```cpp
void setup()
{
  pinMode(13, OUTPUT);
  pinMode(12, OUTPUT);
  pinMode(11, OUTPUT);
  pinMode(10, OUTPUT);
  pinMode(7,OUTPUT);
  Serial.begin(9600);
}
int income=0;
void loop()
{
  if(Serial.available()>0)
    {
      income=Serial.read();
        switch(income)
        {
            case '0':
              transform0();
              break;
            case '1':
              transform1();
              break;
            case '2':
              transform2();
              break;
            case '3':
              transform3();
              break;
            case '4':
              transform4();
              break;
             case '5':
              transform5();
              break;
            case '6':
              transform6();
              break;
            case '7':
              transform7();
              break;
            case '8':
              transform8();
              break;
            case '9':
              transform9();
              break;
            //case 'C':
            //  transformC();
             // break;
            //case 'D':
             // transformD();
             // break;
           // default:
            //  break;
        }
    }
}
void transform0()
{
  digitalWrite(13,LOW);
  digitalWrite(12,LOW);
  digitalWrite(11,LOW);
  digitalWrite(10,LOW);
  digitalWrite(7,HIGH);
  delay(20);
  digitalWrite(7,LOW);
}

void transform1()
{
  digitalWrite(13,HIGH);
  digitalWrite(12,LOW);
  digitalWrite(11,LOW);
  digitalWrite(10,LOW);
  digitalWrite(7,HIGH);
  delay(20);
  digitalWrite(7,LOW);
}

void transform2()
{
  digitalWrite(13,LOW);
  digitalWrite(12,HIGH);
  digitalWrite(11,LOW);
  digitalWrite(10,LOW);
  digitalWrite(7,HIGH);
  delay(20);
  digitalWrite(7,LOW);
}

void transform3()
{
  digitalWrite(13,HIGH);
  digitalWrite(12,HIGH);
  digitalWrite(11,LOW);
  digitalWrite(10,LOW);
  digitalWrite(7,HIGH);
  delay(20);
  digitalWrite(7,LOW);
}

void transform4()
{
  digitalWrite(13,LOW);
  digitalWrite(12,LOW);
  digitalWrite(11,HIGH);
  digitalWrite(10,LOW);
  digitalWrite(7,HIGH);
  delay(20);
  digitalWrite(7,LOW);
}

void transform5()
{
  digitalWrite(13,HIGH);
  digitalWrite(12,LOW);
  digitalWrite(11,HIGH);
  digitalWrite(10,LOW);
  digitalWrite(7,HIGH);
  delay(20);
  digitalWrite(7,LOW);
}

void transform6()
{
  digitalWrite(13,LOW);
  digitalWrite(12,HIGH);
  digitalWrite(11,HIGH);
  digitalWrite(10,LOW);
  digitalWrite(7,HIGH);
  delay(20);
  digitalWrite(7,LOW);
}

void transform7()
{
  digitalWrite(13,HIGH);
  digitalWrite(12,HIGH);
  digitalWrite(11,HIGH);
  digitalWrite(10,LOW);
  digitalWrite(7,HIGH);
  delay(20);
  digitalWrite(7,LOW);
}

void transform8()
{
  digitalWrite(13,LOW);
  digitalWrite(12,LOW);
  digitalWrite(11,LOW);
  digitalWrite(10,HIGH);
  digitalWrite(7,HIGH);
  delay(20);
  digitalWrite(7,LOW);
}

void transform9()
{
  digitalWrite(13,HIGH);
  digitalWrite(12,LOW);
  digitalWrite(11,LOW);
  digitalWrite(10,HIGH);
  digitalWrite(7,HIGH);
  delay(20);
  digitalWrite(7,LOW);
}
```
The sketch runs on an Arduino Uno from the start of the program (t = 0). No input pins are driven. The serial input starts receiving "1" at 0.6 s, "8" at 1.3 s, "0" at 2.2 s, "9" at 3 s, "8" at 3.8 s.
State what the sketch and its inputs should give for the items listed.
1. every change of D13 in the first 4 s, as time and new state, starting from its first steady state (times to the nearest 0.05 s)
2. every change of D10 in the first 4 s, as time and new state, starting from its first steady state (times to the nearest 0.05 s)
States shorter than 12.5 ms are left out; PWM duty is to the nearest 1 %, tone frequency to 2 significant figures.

0 s low; 0.6 s high; 1.3 s low; 3 s high; 3.8 s low
0 s low; 1.3 s high; 2.2 s low; 3 s high
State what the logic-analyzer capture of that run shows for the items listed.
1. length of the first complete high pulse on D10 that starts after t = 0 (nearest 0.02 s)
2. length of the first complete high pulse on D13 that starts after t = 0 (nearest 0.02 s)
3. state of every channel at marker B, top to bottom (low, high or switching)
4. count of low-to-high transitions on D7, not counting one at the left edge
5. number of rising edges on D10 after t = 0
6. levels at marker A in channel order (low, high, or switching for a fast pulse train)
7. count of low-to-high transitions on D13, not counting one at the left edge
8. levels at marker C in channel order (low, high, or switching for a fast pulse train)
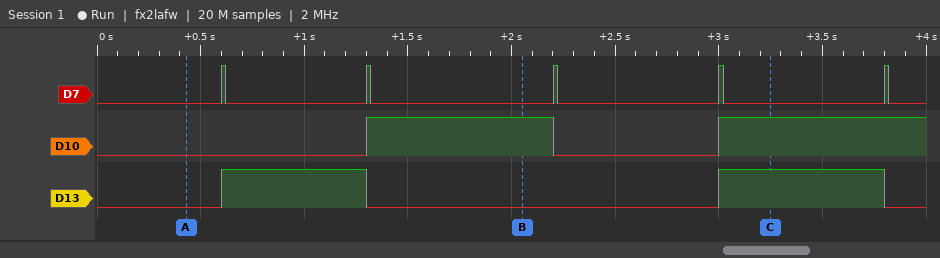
0.90 s
0.70 s
D7 low, D10 high, D13 low
5
2
D7 low, D10 low, D13 low
2
D7 low, D10 high, D13 high
